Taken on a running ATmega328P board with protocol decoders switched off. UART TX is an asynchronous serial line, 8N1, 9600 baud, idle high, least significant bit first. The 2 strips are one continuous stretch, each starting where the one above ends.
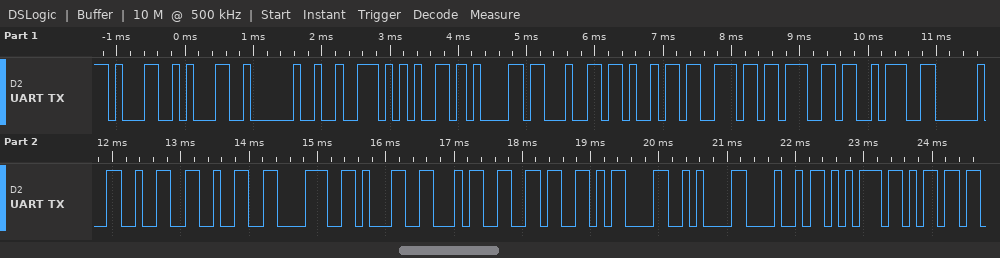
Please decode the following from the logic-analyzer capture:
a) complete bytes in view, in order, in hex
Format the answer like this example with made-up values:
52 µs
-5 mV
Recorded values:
0x31 0x31 0x20 0x72 0x65 0x61 0x64 0x69 0x6E 0x67 0x3A 0x20 0x32 0x32 0x38 0x31 0x34 0x36 0x0D 0x0A 0x48 0x75 0x6D
